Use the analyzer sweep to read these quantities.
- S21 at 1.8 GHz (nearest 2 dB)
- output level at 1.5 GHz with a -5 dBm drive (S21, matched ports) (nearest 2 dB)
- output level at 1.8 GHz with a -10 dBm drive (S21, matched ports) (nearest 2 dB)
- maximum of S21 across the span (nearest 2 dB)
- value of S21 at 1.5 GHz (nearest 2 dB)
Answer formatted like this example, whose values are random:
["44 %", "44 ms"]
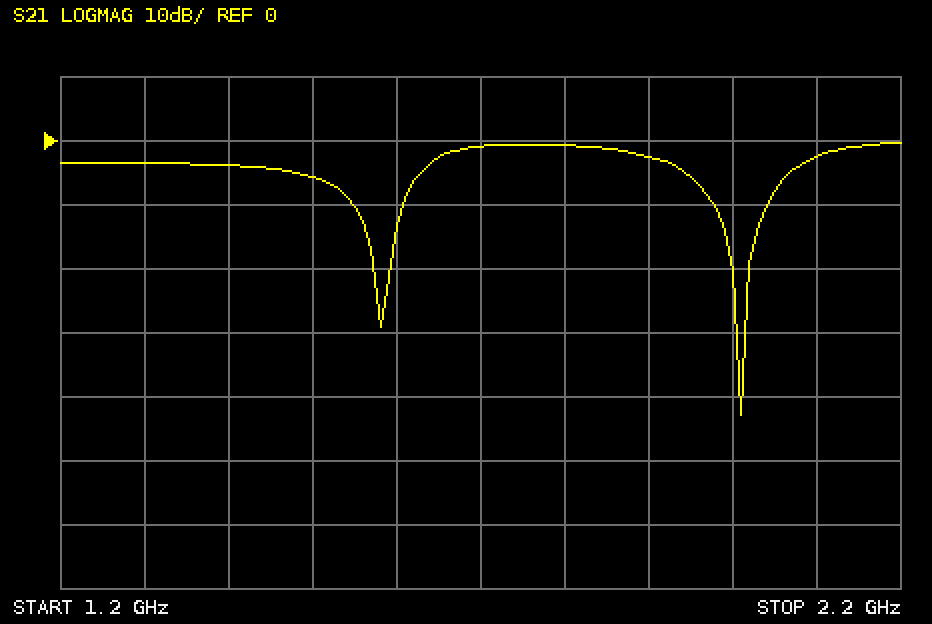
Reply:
["0 dB", "-10 dBm", "-10 dBm", "0 dB", "-6 dB"]
